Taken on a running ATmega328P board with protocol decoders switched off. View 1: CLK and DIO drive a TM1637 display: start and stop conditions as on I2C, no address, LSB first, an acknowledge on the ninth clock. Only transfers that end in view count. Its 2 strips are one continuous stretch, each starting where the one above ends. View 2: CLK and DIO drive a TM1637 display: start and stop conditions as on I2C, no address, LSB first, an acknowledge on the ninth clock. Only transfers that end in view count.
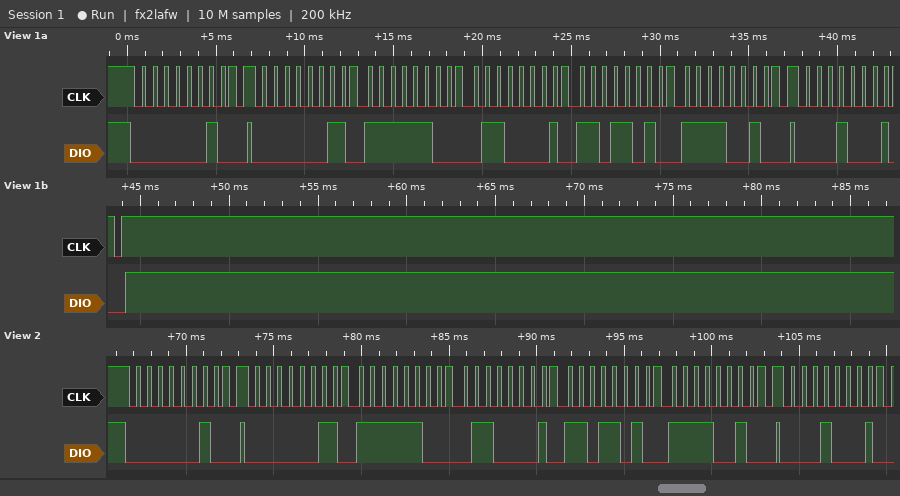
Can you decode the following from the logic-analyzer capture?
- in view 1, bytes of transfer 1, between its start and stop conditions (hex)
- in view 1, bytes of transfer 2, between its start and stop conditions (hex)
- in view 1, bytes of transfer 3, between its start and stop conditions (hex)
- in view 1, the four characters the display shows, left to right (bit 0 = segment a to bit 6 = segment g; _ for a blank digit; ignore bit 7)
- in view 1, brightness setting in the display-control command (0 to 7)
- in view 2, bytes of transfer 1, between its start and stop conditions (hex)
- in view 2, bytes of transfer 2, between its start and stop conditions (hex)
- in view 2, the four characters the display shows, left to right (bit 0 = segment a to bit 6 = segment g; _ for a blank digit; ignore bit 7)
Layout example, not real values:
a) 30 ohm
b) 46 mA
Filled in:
a) 40
b) C0 3F 86 5B 4F
c) 88
d) 0123
e) 0
f) 40
g) C0 3F 86 5B 4F
h) 0123
